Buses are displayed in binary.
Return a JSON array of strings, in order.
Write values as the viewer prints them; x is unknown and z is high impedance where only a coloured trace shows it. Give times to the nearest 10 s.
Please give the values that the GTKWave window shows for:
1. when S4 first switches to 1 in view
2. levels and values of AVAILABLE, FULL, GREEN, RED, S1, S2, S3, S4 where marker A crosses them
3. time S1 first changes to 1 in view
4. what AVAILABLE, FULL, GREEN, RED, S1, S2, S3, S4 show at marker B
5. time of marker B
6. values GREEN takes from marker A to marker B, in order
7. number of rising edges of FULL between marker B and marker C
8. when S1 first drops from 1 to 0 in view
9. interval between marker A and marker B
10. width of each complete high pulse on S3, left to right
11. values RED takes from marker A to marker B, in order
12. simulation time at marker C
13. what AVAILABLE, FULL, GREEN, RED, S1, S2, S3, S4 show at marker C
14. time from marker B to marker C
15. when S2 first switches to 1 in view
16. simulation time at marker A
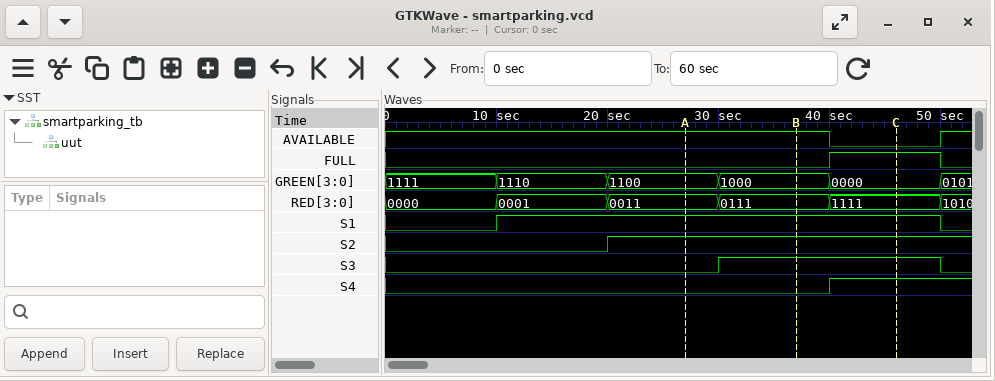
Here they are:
["40 s", "AVAILABLE=1, FULL=0, GREEN=1100, RED=0011, S1=1, S2=1, S3=0, S4=0", "10 s", "AVAILABLE=1, FULL=0, GREEN=1000, RED=0111, S1=1, S2=1, S3=1, S4=0", "40 s", "1100, 1000", "1", "50 s", "10 s", "20 s", "0011, 0111", "50 s", "AVAILABLE=0, FULL=1, GREEN=0000, RED=1111, S1=1, S2=1, S3=1, S4=1", "10 s", "20 s", "30 s"]
